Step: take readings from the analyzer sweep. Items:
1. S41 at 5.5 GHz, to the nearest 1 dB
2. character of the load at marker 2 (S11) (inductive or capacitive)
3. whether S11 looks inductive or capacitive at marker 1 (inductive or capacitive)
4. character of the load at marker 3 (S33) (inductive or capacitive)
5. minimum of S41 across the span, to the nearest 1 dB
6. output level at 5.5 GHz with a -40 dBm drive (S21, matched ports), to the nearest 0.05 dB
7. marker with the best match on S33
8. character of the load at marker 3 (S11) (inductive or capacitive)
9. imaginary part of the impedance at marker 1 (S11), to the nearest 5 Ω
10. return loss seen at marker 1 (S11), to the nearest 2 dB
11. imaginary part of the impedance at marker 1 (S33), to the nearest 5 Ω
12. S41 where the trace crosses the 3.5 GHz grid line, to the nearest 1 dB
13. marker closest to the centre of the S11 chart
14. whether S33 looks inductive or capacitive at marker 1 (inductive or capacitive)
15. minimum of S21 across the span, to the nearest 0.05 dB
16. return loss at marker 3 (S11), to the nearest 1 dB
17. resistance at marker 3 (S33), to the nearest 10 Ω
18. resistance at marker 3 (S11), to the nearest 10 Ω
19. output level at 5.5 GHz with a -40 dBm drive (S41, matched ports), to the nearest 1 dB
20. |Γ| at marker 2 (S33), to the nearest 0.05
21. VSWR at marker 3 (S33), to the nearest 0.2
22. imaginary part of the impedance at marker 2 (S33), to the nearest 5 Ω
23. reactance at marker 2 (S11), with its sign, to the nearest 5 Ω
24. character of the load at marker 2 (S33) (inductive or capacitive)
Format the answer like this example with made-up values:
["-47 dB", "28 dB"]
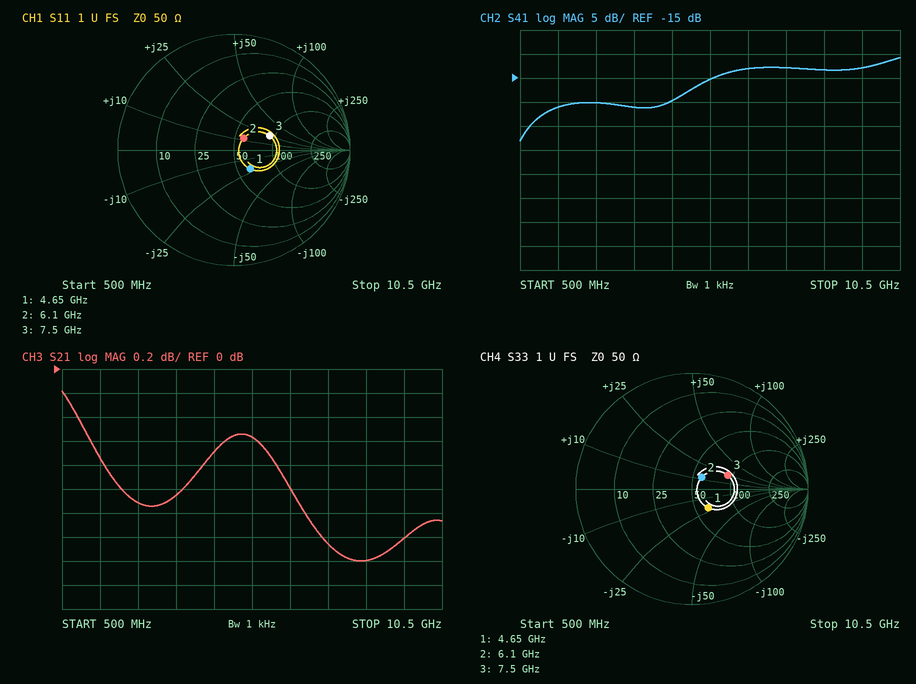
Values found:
["-15 dB", "inductive", "capacitive", "inductive", "-28 dB", "-40.55 dBm", "marker 2", "inductive", "-20 Ω", "14 dB", "-20 Ω", "-21 dB", "marker 2", "capacitive", "-1.60 dB", "10 dB", "90 Ω", "90 Ω", "-55 dBm", "0.15", "2.0", "+10 Ω", "+10 Ω", "inductive"]
